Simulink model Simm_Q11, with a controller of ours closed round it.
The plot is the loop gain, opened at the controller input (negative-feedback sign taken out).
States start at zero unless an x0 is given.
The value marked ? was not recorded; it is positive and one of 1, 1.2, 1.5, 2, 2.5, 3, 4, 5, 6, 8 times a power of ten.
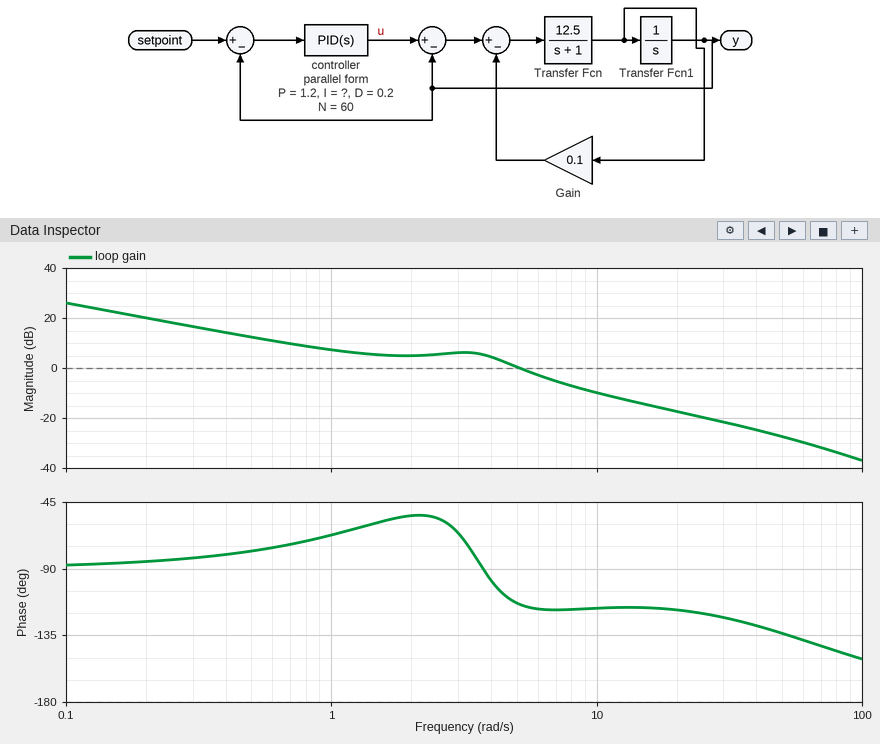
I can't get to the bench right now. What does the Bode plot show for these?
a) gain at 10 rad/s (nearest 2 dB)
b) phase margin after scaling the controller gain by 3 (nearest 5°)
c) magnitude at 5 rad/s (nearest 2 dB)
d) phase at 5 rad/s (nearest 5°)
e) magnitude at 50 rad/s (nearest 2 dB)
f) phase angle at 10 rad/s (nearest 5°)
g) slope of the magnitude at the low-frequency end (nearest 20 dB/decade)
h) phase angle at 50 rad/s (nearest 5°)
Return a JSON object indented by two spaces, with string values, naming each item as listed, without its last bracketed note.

{
  "gain at 10 rad/s": "-10 dB",
  "phase margin after scaling the controller gain by 3": "65°",
  "magnitude at 5 rad/s": "0 dB",
  "phase at 5 rad/s": "-115°",
  "magnitude at 50 rad/s": "-28 dB",
  "phase angle at 10 rad/s": "-115°",
  "slope of the magnitude at the low-frequency end": "-20 dB/decade",
  "phase angle at 50 rad/s": "-135°"
}
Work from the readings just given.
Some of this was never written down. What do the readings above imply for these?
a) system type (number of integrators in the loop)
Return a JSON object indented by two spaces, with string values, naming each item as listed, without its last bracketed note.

{
  "system type": "1"
}
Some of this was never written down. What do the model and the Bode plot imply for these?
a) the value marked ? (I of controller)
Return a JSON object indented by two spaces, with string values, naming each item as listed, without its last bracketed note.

{
  "the value marked ?": "2"
}
